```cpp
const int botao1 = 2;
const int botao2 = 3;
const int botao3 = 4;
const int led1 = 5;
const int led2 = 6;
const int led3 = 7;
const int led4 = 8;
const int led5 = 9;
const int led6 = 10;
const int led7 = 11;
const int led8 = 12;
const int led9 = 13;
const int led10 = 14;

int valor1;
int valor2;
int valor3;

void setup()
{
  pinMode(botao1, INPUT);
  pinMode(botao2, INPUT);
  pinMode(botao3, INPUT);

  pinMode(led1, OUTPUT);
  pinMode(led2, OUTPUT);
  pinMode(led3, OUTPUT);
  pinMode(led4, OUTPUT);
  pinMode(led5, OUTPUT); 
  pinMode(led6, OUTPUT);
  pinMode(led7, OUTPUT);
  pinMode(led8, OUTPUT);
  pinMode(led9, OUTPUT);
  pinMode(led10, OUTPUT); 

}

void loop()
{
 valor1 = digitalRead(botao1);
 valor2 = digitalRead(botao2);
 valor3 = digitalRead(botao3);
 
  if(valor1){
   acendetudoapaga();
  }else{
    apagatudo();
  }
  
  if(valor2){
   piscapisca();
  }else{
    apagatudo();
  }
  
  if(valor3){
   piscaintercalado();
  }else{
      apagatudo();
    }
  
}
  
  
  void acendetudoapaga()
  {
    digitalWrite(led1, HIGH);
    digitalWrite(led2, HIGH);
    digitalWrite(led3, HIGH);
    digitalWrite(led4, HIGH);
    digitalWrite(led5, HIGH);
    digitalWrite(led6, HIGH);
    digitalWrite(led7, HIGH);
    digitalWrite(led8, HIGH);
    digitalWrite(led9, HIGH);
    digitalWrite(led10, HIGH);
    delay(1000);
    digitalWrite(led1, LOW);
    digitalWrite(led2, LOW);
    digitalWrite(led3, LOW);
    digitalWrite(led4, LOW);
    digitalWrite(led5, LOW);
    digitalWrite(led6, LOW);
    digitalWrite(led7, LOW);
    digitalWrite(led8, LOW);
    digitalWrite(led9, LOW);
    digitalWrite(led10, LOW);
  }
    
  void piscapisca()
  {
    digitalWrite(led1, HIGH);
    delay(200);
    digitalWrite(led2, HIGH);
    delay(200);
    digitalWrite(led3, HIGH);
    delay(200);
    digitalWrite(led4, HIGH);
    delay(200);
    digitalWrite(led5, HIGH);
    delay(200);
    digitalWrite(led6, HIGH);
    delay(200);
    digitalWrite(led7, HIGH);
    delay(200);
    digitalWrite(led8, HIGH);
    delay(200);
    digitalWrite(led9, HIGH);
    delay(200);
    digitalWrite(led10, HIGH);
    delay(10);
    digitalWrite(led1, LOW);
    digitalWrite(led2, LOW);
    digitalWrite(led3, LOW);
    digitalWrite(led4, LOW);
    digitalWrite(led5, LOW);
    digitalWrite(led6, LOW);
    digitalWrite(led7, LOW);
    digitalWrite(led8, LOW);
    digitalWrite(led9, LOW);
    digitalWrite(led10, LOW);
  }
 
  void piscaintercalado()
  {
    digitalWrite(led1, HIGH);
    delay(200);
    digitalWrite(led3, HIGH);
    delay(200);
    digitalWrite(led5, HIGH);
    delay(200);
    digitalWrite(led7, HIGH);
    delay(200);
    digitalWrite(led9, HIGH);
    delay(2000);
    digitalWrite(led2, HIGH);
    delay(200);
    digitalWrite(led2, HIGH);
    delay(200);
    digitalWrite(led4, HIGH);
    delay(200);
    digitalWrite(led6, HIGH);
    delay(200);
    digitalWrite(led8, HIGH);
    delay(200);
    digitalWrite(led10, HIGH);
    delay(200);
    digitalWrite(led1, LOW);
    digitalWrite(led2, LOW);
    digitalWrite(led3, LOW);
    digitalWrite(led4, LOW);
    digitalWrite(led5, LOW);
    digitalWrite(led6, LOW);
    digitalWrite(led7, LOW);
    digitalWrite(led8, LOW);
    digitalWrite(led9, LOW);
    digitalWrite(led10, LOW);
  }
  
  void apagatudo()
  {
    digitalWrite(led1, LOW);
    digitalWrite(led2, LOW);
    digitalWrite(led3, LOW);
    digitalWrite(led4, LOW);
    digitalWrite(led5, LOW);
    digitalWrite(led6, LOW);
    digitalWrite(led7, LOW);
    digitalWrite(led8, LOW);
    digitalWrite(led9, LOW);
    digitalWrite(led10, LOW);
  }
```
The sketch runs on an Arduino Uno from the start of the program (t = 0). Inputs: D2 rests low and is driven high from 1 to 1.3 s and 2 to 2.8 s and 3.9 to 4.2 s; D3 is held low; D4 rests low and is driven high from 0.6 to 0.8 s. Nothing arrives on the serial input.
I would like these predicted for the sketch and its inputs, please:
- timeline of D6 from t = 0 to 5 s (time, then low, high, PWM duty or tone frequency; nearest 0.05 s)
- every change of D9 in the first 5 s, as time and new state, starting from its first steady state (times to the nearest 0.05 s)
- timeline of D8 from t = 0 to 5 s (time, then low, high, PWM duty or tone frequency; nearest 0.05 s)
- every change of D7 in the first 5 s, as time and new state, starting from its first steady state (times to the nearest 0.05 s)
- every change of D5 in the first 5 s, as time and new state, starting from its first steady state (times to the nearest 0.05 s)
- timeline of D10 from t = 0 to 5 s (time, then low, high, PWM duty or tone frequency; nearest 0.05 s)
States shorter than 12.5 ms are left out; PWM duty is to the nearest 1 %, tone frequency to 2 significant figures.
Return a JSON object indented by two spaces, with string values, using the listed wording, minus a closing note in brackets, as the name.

{
  "timeline of D6 from t = 0 to 5 s": "0 s low; 3.4 s high; 4.6 s low",
  "every change of D9 in the first 5 s, as time and new state, starting from its first steady state": "0 s low; 1 s high; 4.6 s low",
  "timeline of D8 from t = 0 to 5 s": "0 s low; 3.8 s high; 4.6 s low",
  "every change of D7 in the first 5 s, as time and new state, starting from its first steady state": "0 s low; 0.8 s high; 4.6 s low",
  "every change of D5 in the first 5 s, as time and new state, starting from its first steady state": "0 s low; 0.6 s high; 4.6 s low",
  "timeline of D10 from t = 0 to 5 s": "0 s low; 4 s high; 4.6 s low"
}
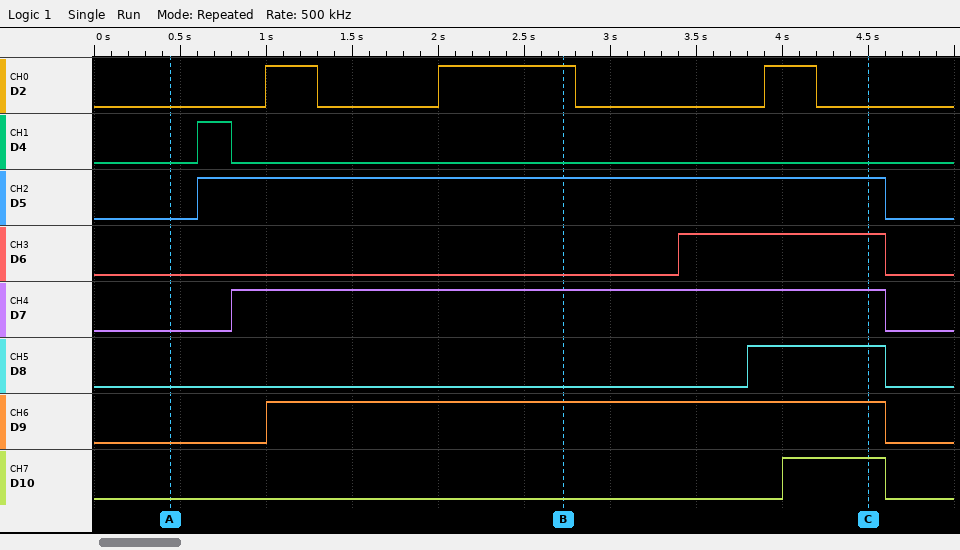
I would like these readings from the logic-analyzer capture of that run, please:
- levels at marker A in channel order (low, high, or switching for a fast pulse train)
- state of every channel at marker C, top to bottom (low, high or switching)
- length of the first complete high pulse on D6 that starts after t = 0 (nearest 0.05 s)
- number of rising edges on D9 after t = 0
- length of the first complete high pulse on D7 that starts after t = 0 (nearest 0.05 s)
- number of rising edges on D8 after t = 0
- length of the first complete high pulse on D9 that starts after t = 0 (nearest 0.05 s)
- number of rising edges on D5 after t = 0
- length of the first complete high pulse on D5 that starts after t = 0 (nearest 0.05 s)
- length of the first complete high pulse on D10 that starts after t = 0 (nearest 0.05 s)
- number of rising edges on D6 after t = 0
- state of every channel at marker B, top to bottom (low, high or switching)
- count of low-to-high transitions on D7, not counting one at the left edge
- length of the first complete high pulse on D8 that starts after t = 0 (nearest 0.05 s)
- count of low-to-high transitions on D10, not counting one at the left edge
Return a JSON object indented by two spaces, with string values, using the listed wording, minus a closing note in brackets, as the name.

{
  "levels at marker A in channel order": "D2 low, D4 low, D5 low, D6 low, D7 low, D8 low, D9 low, D10 low",
  "state of every channel at marker C, top to bottom": "D2 low, D4 low, D5 high, D6 high, D7 high, D8 high, D9 high, D10 high",
  "length of the first complete high pulse on D6 that starts after t = 0": "1.20 s",
  "number of rising edges on D9 after t = 0": "1",
  "length of the first complete high pulse on D7 that starts after t = 0": "3.80 s",
  "number of rising edges on D8 after t = 0": "1",
  "length of the first complete high pulse on D9 that starts after t = 0": "3.60 s",
  "number of rising edges on D5 after t = 0": "1",
  "length of the first complete high pulse on D5 that starts after t = 0": "4.00 s",
  "length of the first complete high pulse on D10 that starts after t = 0": "0.60 s",
  "number of rising edges on D6 after t = 0": "1",
  "state of every channel at marker B, top to bottom": "D2 high, D4 low, D5 high, D6 low, D7 high, D8 low, D9 high, D10 low",
  "count of low-to-high transitions on D7, not counting one at the left edge": "1",
  "length of the first complete high pulse on D8 that starts after t = 0": "0.80 s",
  "count of low-to-high transitions on D10, not counting one at the left edge": "1"
}
